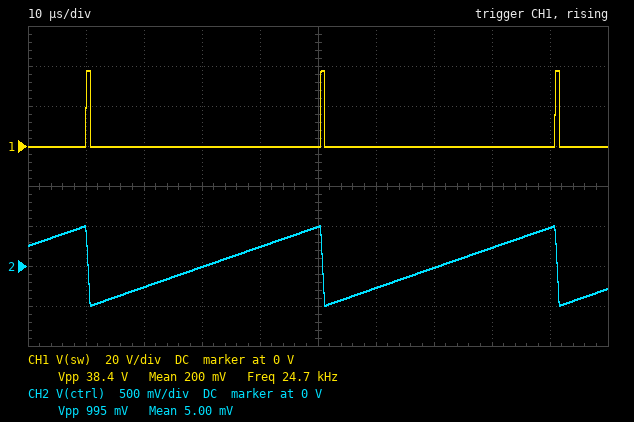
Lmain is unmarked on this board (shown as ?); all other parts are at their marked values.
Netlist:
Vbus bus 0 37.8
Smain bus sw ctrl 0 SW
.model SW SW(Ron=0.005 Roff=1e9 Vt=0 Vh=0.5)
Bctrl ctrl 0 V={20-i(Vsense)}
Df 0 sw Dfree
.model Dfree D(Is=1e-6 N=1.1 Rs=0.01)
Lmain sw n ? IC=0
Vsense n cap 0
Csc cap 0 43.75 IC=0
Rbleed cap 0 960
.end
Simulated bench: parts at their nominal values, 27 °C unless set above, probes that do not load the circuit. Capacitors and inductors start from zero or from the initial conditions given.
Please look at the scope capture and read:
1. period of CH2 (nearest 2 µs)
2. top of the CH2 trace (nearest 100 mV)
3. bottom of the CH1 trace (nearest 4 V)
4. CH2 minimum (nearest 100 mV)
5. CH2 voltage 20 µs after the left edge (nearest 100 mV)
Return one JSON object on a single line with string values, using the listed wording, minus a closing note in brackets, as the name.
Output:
{"period of CH2": "40 µs", "top of the CH2 trace": "500 mV", "bottom of the CH1 trace": "0 V", "CH2 minimum": "-500 mV", "CH2 voltage 20 µs after the left edge": "-300 mV"}
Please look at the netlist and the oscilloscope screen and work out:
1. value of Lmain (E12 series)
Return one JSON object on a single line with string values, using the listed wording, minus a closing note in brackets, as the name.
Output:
{"value of Lmain": "27 µH"}
